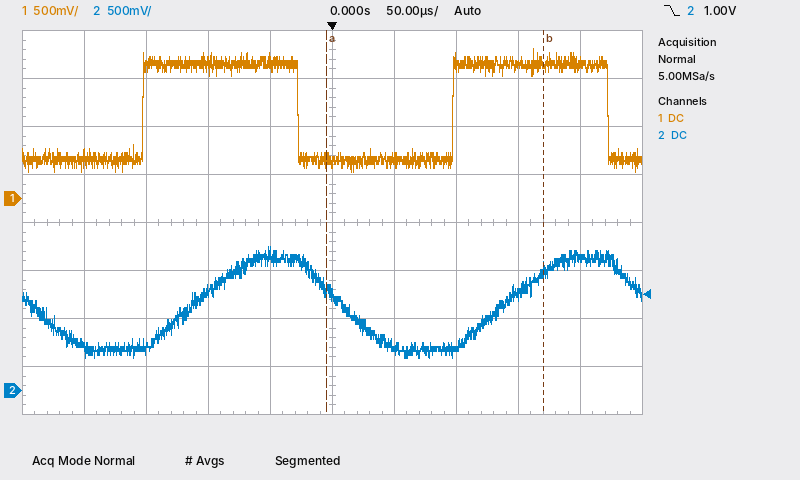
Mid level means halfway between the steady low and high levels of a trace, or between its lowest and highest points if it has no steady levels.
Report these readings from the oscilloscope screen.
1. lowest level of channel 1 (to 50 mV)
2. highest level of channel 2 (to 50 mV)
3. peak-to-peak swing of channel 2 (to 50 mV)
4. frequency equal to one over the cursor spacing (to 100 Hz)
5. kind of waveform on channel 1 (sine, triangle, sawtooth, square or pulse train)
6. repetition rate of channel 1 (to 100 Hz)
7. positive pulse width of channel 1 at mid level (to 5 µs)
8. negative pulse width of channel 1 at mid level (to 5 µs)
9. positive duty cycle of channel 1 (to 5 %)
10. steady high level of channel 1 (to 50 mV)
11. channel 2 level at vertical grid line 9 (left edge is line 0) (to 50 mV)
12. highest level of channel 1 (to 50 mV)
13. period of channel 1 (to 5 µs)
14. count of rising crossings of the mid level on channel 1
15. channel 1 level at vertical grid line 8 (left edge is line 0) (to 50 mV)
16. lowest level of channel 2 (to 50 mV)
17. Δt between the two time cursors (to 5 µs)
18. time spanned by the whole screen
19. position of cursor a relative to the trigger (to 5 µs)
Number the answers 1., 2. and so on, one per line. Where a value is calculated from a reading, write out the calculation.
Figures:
1. 300 mV
2. 1.50 V
3. 1.50 V − (350 mV) = 1.15 V
4. 1 / 175 µs ≈ 5.7 kHz
5. square
6. 1 / 250 µs ≈ 4.0 kHz
7. 125 µs
8. 125 µs
9. 125 µs / 250 µs ≈ 50 %
10. 1.40 V
11. 1.40 V
12. 1.55 V
13. 250 µs
14. 2
15. 1.40 V
16. 350 mV
17. 175 µs
18. 500 µs
19. -5 µs
